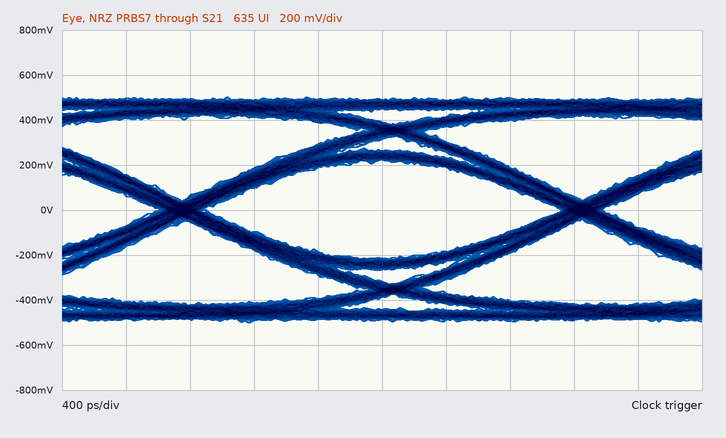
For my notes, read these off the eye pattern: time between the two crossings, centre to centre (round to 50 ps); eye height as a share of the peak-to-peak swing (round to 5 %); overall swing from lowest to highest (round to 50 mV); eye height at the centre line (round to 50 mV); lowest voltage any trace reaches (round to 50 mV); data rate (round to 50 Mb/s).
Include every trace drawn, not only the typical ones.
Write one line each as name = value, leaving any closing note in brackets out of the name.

time between the two crossings, centre to centre = 2.50 ns
eye height as a share of the peak-to-peak swing = 45 %
overall swing from lowest to highest = 1.00 V
eye height at the centre line = 450 mV
lowest voltage any trace reaches = -500 mV
data rate = 400 Mb/s
